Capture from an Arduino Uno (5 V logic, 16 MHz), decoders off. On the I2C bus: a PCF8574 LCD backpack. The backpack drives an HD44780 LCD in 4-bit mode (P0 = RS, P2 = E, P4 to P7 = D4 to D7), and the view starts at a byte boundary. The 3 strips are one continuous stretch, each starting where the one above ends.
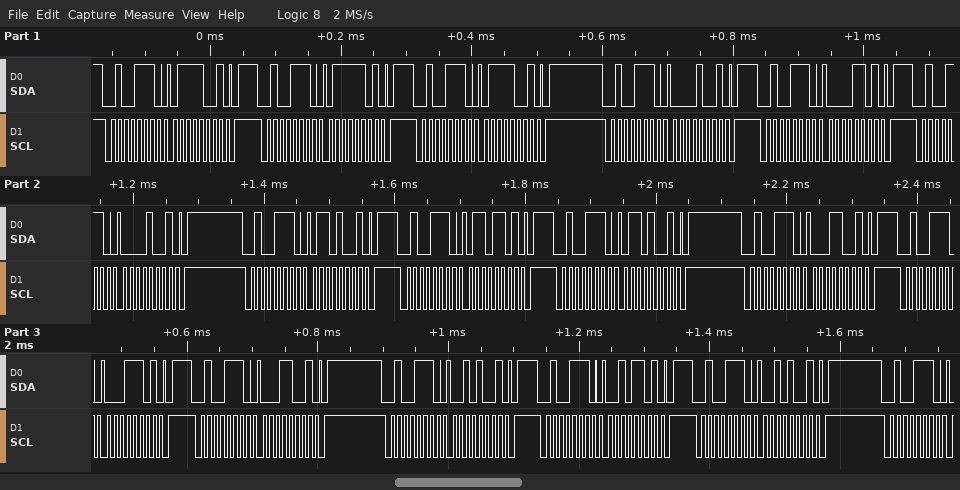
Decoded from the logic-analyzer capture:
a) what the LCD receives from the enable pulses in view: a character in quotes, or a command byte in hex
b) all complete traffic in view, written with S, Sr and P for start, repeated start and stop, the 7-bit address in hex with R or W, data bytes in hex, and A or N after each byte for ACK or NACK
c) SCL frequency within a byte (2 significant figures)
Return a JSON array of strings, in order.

["'p' 'a'", "S 27W A 79 A P S 27W A 7D A P S 27W A 79 A P S 27W A 09 A P S 27W A 0D A P S 27W A 09 A P S 27W A 69 A P S 27W A 6D A P S 27W A 69 A P S 27W A 19 A P S 27W A 1D A P S 27W A 19 A P S 27W A 29 A P S 27W A 2D A P S 27W A 29 A P S 27W A", "100 kHz"]
